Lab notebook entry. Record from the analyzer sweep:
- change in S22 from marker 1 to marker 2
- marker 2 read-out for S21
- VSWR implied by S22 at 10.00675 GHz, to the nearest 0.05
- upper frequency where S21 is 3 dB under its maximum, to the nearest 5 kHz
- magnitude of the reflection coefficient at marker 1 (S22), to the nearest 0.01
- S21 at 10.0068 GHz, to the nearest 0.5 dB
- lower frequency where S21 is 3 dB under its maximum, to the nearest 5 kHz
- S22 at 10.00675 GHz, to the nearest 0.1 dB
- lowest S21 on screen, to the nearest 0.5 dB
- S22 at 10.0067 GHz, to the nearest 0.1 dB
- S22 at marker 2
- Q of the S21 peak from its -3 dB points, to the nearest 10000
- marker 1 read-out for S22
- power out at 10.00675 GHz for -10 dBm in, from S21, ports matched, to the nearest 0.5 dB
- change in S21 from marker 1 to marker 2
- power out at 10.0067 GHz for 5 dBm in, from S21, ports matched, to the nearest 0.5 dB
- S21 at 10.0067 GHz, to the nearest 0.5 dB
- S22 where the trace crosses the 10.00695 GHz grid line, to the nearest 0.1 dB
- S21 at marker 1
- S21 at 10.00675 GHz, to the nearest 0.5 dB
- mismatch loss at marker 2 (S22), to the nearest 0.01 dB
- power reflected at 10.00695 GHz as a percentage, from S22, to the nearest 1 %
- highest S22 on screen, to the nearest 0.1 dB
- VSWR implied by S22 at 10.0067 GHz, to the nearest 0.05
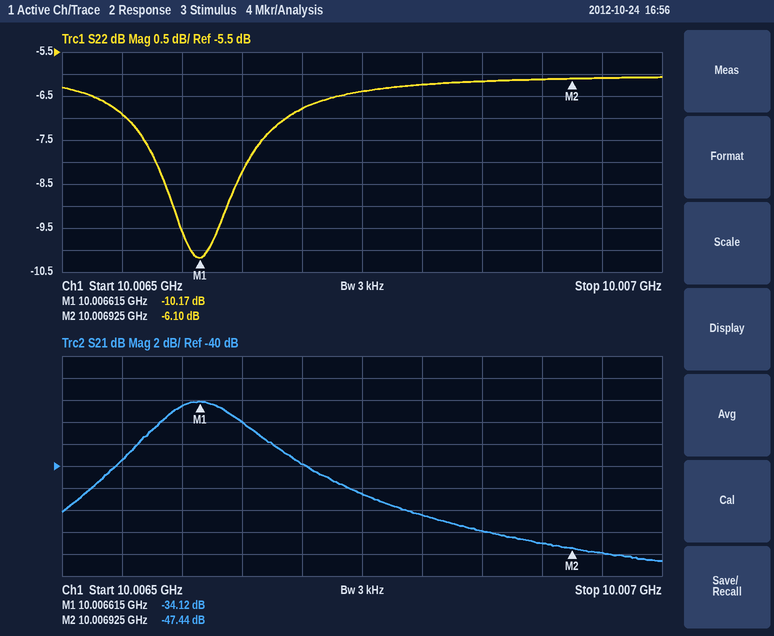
4.07 dB
-47.44 dB
2.85
10.006665 GHz
0.31
-44.5 dB
10.006570 GHz
-6.4 dB
-48.5 dB
-6.8 dB
-6.10 dB
110000
-10.17 dB
-52.5 dBm
-13.32 dB
-35.0 dBm
-40.0 dB
-6.1 dB
-34.12 dB
-42.5 dB
1.22 dB
25 %
-6.1 dB
2.70
